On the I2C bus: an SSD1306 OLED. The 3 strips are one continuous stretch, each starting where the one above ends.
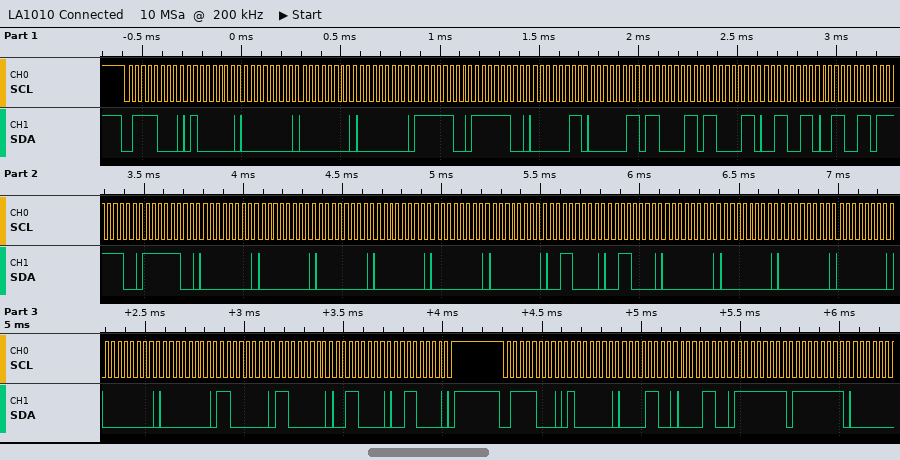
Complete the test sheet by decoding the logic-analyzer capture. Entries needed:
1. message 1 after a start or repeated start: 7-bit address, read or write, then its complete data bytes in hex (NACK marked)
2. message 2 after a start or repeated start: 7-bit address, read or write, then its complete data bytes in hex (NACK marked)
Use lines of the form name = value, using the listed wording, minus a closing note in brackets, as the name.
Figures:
message 1 after a start or repeated start: 7-bit address, read or write, then its complete data bytes in hex = 0x3C write: 40 00 00 00 FC FC 03 03 C3 C3 33 33 FC FC 00 00 00 00 00 00 30 30 00 00 00 00 00 00 C0 C0 30 30
message 2 after a start or repeated start: 7-bit address, read or write, then its complete data bytes in hex = 0x3C write: 40 0C 0C FF FF
